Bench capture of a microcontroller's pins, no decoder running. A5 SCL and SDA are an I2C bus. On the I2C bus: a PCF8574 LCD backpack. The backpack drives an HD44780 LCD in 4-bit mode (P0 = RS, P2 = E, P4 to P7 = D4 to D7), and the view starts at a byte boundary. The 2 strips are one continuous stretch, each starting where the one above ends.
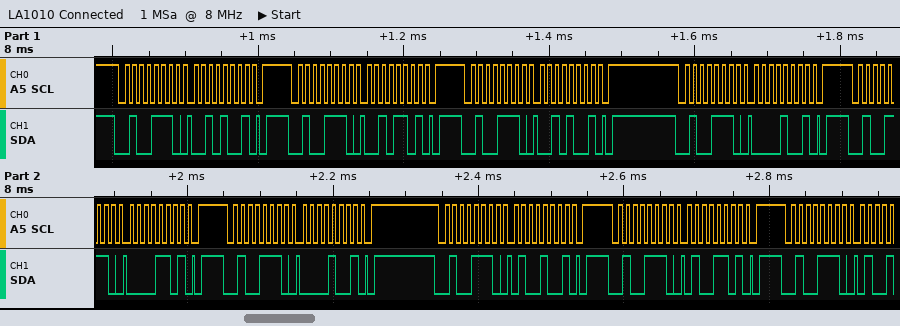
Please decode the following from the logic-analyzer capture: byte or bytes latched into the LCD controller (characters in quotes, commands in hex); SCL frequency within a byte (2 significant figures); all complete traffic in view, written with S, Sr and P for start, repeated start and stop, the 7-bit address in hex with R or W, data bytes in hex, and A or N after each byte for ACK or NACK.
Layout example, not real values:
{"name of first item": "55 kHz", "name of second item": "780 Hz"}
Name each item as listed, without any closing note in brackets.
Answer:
{"byte or bytes latched into the LCD controller": "' '", "SCL frequency within a byte": "100 kHz", "all complete traffic in view, written with S, Sr and P for start, repeated start and stop, the 7-bit address in hex with R or W, data bytes in hex, and A or N after each byte for ACK or NACK": "S 27W A 29 A P S 27W A 2D A P S 27W A 29 A P S 27W A 09 A P S 27W A 0D A P S 27W A 09 A P S 27W A 49 A P S 27W A 4D A P S 27W A"}
